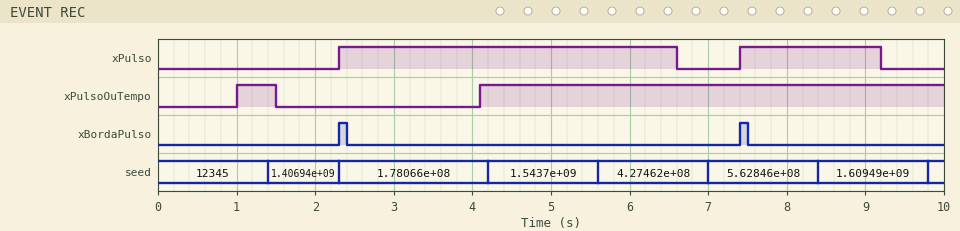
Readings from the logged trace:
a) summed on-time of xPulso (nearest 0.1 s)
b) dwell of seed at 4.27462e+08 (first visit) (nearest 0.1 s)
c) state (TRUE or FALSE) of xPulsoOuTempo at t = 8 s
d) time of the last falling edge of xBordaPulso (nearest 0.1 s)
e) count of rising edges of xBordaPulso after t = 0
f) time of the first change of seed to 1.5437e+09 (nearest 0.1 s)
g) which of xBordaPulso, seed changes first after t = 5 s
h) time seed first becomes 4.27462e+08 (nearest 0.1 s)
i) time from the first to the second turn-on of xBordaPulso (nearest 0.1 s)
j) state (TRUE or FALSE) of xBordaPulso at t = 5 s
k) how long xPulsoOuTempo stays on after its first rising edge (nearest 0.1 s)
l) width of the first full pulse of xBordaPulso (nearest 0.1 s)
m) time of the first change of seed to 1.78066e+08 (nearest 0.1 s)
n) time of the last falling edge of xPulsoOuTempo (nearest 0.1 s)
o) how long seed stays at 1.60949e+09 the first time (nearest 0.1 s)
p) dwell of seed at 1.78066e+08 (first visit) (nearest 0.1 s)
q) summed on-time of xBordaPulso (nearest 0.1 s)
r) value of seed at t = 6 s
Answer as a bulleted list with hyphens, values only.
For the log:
- 6.1 s
- 1.4 s
- TRUE
- 7.5 s
- 2
- 4.2 s
- seed
- 5.6 s
- 5.1 s
- FALSE
- 0.5 s
- 0.1 s
- 2.3 s
- 1.5 s
- 1.4 s
- 1.9 s
- 0.2 s
- 4.27462e+08
